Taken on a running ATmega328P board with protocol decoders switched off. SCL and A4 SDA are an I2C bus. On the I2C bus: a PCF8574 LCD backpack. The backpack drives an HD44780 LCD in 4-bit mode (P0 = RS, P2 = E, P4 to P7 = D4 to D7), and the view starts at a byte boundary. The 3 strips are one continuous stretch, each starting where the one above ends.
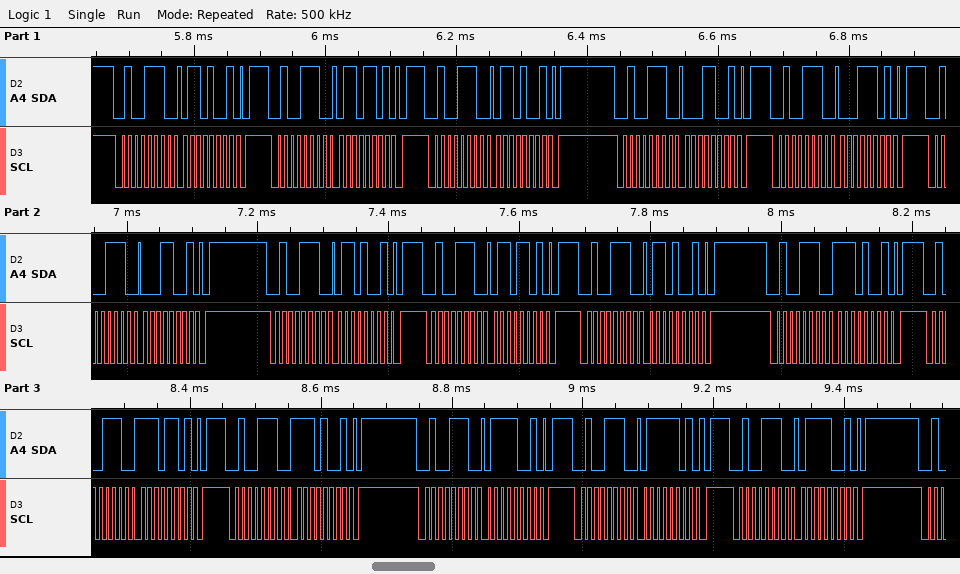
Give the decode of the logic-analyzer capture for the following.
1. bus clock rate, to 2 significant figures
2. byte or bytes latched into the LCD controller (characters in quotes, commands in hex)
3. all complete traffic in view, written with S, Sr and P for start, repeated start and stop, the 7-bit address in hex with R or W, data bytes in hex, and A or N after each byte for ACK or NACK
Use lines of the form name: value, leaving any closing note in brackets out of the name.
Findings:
bus clock rate, to 2 significant figures: 100 kHz
byte or bytes latched into the LCD controller: 'a' 'n'
all complete traffic in view, written with S, Sr and P for start, repeated start and stop, the 7-bit address in hex with R or W, data bytes in hex, and A or N after each byte for ACK or NACK: S 27W A 69 A P S 27W A 6D A P S 27W A 69 A P S 27W A 19 A P S 27W A 1D A P S 27W A 19 A P S 27W A 69 A P S 27W A 6D A P S 27W A 69 A P S 27W A E9 A P S 27W A ED A P S 27W A E9 A P S 27W A 79 A P S 27W A 7D A P S 27W A 79 A P
